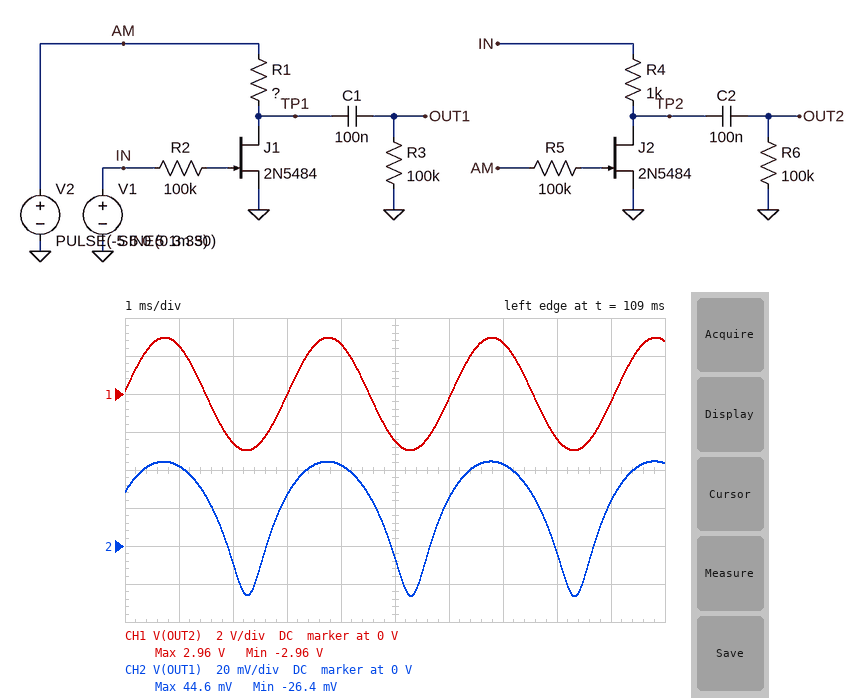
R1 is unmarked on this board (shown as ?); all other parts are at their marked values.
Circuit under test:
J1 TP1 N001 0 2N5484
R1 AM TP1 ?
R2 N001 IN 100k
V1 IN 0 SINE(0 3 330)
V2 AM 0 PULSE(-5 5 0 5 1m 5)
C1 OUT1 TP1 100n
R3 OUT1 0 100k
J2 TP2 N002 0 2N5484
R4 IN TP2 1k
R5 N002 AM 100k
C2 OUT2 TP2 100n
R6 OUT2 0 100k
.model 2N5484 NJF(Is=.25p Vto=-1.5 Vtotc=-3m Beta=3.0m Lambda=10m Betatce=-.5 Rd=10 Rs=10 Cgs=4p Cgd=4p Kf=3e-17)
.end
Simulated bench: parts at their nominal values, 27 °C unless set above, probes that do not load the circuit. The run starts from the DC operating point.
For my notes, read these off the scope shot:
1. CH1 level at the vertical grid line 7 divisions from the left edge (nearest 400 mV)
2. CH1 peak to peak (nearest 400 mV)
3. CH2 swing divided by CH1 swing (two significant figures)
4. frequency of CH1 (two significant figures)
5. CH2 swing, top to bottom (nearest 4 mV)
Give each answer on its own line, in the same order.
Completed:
2.8 V
6.0 V
0.012
330 Hz
72 mV
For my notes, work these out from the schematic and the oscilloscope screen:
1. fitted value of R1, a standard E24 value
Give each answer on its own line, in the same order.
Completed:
75 Ω
